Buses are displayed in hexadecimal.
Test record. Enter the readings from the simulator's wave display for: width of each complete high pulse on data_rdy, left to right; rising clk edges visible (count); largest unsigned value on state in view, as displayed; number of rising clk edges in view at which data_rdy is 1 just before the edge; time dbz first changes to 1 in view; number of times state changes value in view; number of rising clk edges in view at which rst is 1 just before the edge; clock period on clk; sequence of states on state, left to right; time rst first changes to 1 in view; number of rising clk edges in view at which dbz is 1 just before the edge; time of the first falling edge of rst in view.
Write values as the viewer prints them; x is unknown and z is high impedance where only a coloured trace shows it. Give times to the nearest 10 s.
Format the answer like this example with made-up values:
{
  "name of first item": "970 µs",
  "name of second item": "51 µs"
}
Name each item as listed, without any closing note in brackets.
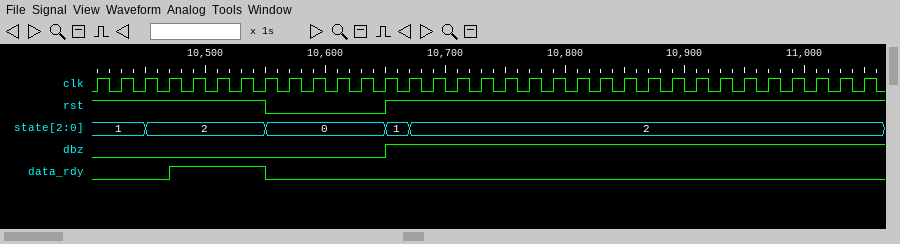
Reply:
{
  "width of each complete high pulse on data_rdy, left to right": "80 s",
  "rising clk edges visible": "33",
  "largest unsigned value on state in view, as displayed": "2",
  "number of rising clk edges in view at which data_rdy is 1 just before the edge": "4",
  "time dbz first changes to 1 in view": "10650 s",
  "number of times state changes value in view": "4",
  "number of rising clk edges in view at which rst is 1 just before the edge": "28",
  "clock period on clk": "20 s",
  "sequence of states on state, left to right": "1, 2, 0, 1, 2",
  "time rst first changes to 1 in view": "10650 s",
  "number of rising clk edges in view at which dbz is 1 just before the edge": "20",
  "time of the first falling edge of rst in view": "10550 s"
}
